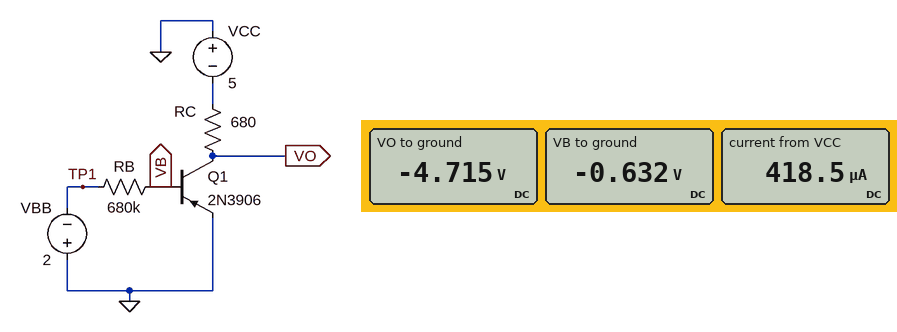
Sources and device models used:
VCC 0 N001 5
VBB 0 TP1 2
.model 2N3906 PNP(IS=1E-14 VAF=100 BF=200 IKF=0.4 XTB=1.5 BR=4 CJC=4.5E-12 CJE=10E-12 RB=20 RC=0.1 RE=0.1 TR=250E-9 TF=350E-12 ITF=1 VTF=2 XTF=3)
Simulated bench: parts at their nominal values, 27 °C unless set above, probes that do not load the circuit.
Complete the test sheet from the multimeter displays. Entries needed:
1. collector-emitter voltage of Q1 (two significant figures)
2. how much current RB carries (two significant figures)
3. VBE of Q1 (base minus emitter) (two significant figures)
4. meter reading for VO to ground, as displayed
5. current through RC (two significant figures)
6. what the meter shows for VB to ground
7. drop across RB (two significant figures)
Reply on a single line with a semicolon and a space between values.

-4.7 V; 2.0 µA; -630 mV; -4.715 V; 420 µA; -0.632 V; 1.4 V
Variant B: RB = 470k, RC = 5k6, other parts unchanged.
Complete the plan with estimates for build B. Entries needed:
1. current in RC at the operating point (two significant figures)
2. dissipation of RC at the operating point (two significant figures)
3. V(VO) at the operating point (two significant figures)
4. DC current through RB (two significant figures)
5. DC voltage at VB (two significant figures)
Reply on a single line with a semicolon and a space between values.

580 µA; 1.9 mW; -1.7 V; 2.9 µA; -640 mV
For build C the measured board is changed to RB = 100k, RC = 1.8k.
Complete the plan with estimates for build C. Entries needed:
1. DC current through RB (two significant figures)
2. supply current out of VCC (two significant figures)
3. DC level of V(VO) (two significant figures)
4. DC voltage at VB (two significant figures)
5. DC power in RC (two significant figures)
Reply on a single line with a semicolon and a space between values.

13 µA; 2.6 mA; -300 mV; -680 mV; 12 mW
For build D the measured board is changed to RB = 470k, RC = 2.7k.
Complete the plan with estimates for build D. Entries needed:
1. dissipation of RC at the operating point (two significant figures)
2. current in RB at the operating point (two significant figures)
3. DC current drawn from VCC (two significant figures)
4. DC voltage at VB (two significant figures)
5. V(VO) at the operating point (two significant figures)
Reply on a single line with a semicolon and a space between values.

950 µW; 2.9 µA; 590 µA; -640 mV; -3.4 V
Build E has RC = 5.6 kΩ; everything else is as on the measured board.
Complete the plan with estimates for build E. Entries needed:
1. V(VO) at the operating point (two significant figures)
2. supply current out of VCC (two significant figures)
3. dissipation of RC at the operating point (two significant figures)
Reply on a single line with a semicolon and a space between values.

-2.7 V; 410 µA; 940 µW
